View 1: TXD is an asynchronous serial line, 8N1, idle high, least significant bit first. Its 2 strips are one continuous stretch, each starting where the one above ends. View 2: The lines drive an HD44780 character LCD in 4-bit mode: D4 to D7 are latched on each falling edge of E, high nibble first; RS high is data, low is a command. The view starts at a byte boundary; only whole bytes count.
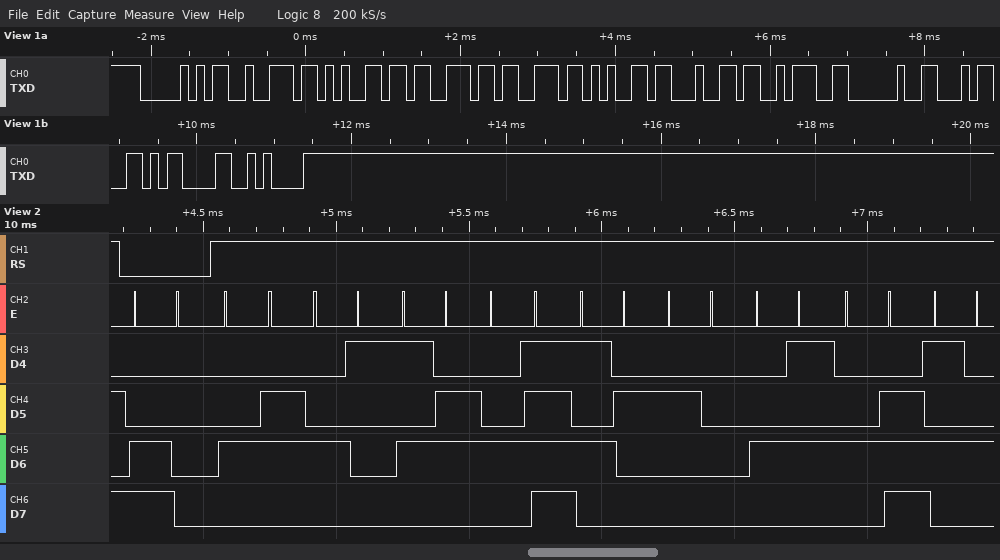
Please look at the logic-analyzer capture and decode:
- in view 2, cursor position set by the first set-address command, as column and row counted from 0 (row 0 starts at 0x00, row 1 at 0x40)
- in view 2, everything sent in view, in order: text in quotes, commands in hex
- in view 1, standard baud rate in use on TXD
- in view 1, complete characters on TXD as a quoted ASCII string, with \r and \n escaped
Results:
column 0, row 1
0xC0 "FAVOR ENT"
9600 baud
"Pressed: 4\r\n"
